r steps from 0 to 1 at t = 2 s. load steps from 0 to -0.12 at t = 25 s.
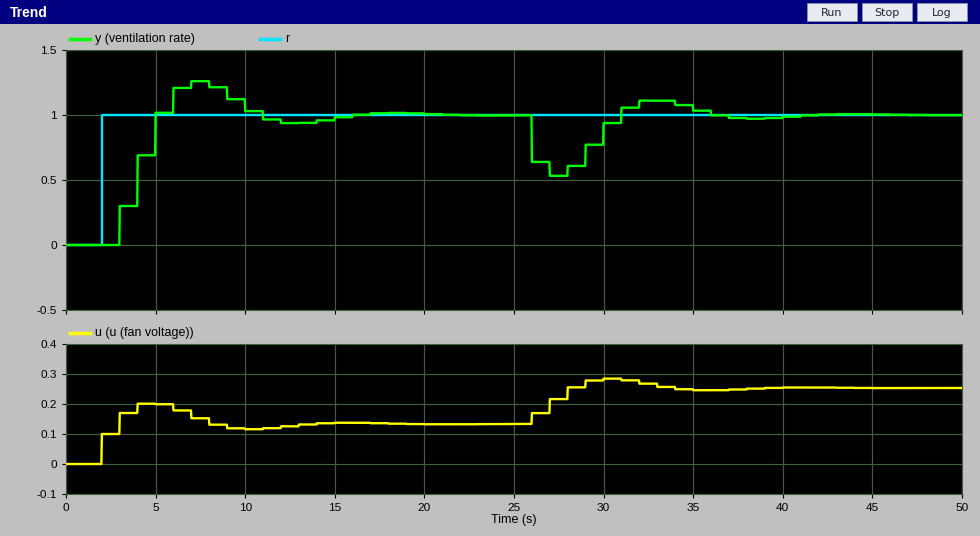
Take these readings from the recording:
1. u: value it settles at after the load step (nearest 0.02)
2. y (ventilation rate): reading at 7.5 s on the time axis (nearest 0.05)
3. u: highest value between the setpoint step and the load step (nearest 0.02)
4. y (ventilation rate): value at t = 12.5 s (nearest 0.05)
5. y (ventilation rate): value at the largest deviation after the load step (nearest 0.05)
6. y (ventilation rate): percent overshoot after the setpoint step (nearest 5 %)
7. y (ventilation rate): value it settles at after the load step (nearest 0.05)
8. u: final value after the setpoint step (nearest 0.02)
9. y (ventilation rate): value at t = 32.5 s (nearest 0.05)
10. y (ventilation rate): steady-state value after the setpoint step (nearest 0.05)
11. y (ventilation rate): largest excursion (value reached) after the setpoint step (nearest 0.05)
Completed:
0.26
1.25
0.20
0.95
0.55
25 %
1.00
0.14
1.10
1.00
1.25
